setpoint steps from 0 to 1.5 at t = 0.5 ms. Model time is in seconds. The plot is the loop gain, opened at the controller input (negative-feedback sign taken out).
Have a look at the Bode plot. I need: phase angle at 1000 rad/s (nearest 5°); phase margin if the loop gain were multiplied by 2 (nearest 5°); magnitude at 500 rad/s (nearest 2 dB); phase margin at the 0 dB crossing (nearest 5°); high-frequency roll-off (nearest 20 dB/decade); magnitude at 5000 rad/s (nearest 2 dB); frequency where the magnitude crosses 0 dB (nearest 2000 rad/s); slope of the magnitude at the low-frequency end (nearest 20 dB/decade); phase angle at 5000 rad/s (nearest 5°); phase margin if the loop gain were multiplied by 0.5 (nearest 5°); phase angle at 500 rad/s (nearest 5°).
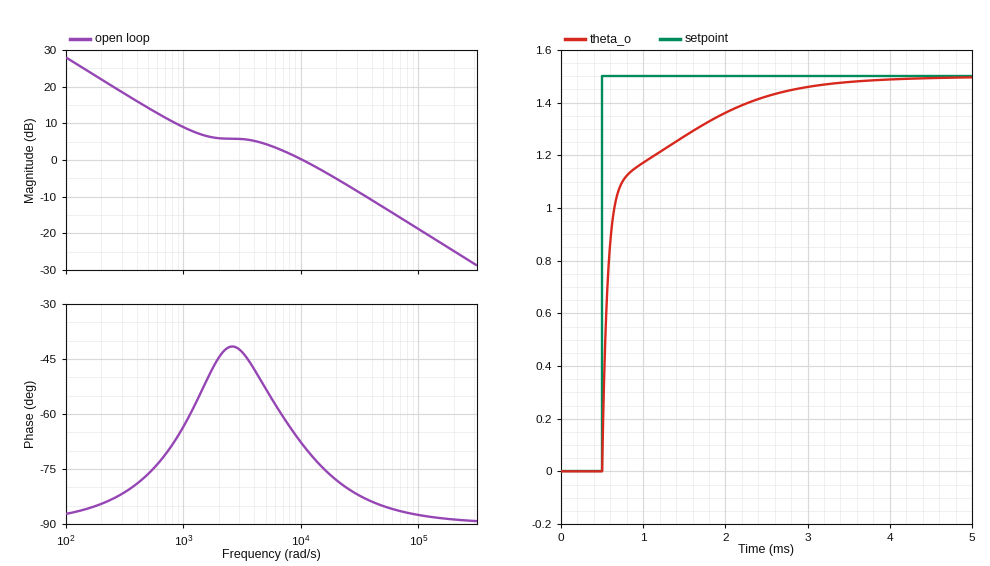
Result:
-65°
100°
14 dB
110°
-20 dB/decade
4 dB
10000 rad/s
-20 dB/decade
-55°
135°
-75°
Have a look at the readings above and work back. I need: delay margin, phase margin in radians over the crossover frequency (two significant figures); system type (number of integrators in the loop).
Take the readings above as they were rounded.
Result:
0.00019 s
1
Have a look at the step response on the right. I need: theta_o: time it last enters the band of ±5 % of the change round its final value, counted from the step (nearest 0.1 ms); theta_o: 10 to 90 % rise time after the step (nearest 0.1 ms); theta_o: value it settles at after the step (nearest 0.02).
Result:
2.0 ms
1.4 ms
1.50
